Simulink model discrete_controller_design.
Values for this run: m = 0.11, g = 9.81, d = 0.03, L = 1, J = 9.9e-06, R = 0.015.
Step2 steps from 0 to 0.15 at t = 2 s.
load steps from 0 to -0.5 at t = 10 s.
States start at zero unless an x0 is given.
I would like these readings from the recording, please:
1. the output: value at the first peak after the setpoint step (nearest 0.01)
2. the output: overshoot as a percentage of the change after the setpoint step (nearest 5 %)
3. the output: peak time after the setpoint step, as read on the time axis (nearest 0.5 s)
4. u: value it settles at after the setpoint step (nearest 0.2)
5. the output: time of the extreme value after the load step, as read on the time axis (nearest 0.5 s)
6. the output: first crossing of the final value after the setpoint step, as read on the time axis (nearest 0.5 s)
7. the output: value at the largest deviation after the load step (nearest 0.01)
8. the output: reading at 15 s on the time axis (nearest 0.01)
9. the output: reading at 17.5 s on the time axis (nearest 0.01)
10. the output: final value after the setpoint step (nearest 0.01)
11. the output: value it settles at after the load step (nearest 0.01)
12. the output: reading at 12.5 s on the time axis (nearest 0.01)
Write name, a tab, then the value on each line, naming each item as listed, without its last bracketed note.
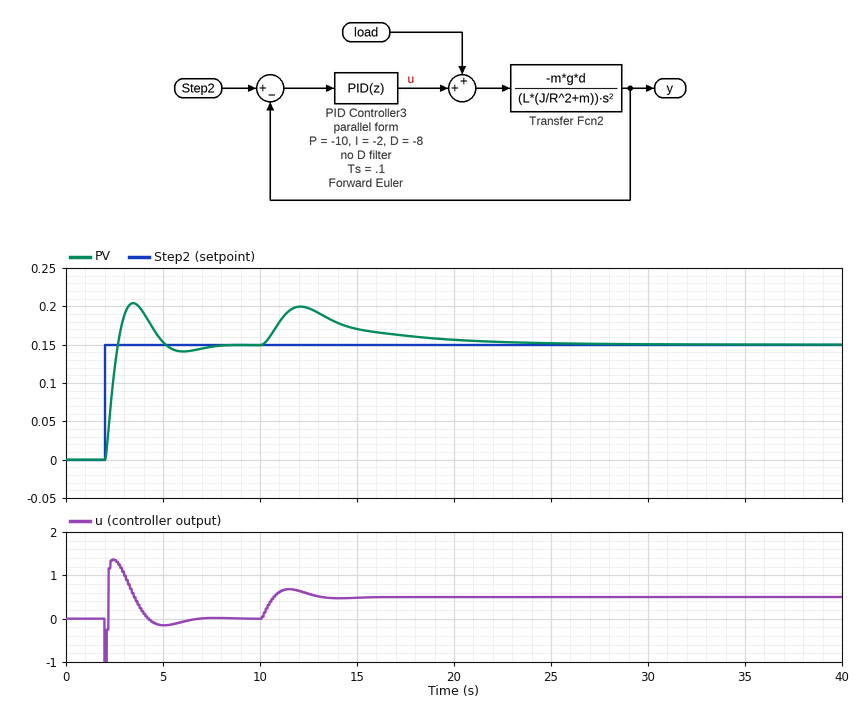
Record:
the output: value at the first peak after the setpoint step	0.20
the output: overshoot as a percentage of the change after the setpoint step	35 %
the output: peak time after the setpoint step, as read on the time axis	3.5 s
u: value it settles at after the setpoint step	0.0
the output: time of the extreme value after the load step, as read on the time axis	12.0 s
the output: first crossing of the final value after the setpoint step, as read on the time axis	2.5 s
the output: value at the largest deviation after the load step	0.20
the output: reading at 15 s on the time axis	0.17
the output: reading at 17.5 s on the time axis	0.16
the output: final value after the setpoint step	0.15
the output: value it settles at after the load step	0.15
the output: reading at 12.5 s on the time axis	0.20
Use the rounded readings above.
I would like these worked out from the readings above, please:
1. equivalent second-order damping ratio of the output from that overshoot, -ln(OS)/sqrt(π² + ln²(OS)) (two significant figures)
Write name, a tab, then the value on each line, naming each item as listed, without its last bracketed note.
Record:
equivalent second-order damping ratio of the output from that overshoot, -ln(OS)/sqrt(π² + ln²(OS))	0.32
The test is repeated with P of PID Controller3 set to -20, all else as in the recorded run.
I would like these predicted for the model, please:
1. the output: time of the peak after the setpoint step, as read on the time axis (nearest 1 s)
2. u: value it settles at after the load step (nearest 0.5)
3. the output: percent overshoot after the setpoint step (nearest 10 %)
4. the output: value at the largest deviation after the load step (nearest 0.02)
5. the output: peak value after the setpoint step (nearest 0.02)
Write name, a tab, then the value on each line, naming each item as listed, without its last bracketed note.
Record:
the output: time of the peak after the setpoint step, as read on the time axis	3 s
u: value it settles at after the load step	0.5
the output: percent overshoot after the setpoint step	50 %
the output: value at the largest deviation after the load step	0.18
the output: peak value after the setpoint step	0.22
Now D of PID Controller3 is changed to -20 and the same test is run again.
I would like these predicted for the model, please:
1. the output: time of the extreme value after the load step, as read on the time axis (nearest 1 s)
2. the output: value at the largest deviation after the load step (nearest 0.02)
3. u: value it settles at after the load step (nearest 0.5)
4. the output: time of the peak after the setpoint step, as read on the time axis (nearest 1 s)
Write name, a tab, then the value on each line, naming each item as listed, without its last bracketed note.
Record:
the output: time of the extreme value after the load step, as read on the time axis	13 s
the output: value at the largest deviation after the load step	0.18
u: value it settles at after the load step	0.5
the output: time of the peak after the setpoint step, as read on the time axis	3 s
